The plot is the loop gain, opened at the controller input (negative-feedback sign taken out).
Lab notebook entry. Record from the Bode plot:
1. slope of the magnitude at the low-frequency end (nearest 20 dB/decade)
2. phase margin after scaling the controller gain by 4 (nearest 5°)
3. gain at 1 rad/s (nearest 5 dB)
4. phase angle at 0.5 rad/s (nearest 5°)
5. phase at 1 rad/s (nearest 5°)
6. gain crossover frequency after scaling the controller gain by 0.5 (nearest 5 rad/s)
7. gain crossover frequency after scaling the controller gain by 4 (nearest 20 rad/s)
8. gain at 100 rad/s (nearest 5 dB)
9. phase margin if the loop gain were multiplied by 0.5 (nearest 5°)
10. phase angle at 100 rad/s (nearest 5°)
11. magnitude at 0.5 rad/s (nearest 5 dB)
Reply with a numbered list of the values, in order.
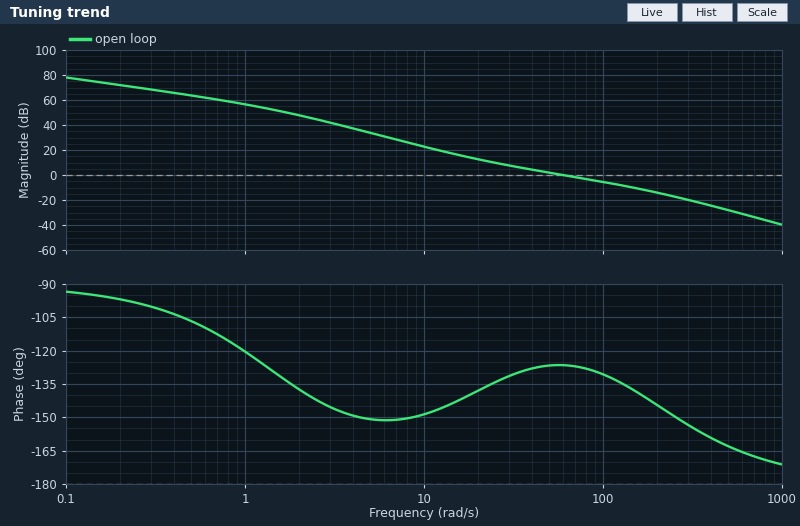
1. -20 dB/decade
2. 40°
3. 55 dB
4. -105°
5. -120°
6. 35 rad/s
7. 180 rad/s
8. -5 dB
9. 50°
10. -130°
11. 65 dB
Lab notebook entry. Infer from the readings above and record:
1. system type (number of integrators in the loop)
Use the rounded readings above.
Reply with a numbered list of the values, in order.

1. 1
